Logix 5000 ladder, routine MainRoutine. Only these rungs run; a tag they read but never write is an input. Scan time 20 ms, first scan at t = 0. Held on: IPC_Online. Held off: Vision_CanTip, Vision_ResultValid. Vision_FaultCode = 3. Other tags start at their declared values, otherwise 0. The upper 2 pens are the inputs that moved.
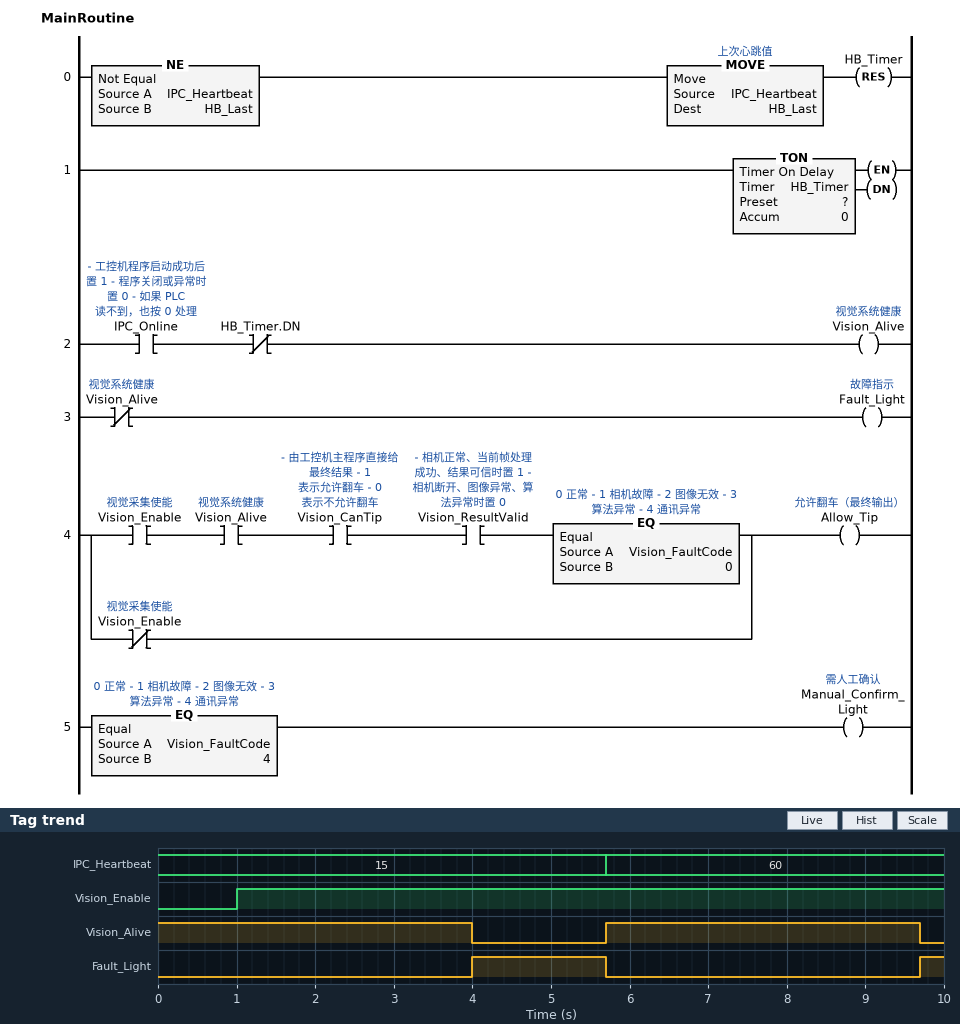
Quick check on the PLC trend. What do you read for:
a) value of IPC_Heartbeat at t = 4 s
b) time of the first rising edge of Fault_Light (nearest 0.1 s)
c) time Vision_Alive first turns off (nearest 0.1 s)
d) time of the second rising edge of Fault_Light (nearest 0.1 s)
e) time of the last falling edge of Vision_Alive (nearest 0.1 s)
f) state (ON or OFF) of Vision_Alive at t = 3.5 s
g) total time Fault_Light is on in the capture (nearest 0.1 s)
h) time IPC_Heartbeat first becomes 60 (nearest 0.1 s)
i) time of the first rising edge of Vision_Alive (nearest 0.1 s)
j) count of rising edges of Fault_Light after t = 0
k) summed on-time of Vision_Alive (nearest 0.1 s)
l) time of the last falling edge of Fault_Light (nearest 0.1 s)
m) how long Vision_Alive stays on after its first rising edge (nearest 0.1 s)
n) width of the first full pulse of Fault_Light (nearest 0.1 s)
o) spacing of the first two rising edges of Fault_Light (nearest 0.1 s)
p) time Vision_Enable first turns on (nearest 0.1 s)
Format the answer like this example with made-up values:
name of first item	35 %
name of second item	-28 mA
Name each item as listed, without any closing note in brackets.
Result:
value of IPC_Heartbeat at t = 4 s	15
time of the first rising edge of Fault_Light	4.0 s
time Vision_Alive first turns off	4.0 s
time of the second rising edge of Fault_Light	9.7 s
time of the last falling edge of Vision_Alive	9.7 s
state (ON or OFF) of Vision_Alive at t = 3.5 s	ON
total time Fault_Light is on in the capture	2.0 s
time IPC_Heartbeat first becomes 60	5.7 s
time of the first rising edge of Vision_Alive	5.7 s
count of rising edges of Fault_Light after t = 0	2
summed on-time of Vision_Alive	8.0 s
time of the last falling edge of Fault_Light	5.7 s
how long Vision_Alive stays on after its first rising edge	4.0 s
width of the first full pulse of Fault_Light	1.7 s
spacing of the first two rising edges of Fault_Light	5.7 s
time Vision_Enable first turns on	1.0 s
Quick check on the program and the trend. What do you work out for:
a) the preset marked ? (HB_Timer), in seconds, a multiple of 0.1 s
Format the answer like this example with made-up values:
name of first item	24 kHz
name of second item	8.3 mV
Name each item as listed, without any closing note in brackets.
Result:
the preset marked ? (HB_Timer), in seconds, a multiple of 0.1 s	4.0 s
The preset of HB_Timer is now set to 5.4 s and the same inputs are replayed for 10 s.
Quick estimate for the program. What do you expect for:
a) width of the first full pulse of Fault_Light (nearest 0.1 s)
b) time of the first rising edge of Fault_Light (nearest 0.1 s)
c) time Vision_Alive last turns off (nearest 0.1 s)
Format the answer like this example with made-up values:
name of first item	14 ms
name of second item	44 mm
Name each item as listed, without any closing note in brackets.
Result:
width of the first full pulse of Fault_Light	0.3 s
time of the first rising edge of Fault_Light	5.4 s
time Vision_Alive last turns off	5.4 s
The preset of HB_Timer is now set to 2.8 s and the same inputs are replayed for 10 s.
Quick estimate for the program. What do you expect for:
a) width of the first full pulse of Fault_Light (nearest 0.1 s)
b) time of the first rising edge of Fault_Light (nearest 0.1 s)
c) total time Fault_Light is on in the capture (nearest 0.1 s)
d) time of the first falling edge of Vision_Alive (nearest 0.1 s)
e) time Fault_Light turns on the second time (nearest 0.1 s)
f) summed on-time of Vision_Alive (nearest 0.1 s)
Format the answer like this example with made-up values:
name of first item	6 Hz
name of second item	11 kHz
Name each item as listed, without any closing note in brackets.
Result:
width of the first full pulse of Fault_Light	2.9 s
time of the first rising edge of Fault_Light	2.8 s
total time Fault_Light is on in the capture	4.4 s
time of the first falling edge of Vision_Alive	2.8 s
time Fault_Light turns on the second time	8.5 s
summed on-time of Vision_Alive	5.6 s
